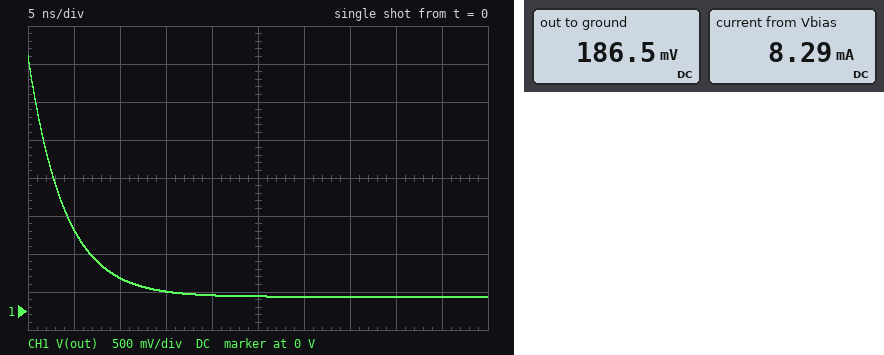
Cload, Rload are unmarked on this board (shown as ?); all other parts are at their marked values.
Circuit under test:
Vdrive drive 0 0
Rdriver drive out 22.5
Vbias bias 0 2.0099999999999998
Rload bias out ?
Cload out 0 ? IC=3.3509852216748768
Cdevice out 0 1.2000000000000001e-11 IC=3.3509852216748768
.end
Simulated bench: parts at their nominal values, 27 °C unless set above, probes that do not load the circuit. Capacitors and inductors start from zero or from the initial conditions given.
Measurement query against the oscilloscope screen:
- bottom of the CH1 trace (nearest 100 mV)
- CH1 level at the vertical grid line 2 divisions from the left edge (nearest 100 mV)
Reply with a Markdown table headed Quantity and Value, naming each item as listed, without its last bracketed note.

| Quantity | Value |
|---|---|
| bottom of the CH1 trace | 200 mV |
| CH1 level at the vertical grid line 2 divisions from the left edge | 400 mV |
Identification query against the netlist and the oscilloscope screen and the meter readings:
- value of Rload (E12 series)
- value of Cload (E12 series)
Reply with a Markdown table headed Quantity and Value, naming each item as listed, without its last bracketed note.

| Quantity | Value |
|---|---|
| value of Rload | 220 Ω |
| value of Cload | 180 pF |
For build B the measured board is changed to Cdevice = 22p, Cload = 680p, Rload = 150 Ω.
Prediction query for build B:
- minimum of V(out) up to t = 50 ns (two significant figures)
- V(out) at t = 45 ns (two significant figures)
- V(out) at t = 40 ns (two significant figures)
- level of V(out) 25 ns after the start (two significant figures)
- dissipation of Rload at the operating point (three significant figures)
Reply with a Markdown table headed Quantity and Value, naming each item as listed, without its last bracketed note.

| Quantity | Value |
|---|---|
| minimum of V(out) up to t = 50 ns | 340 mV |
| V(out) at t = 45 ns | 380 mV |
| V(out) at t = 40 ns | 430 mV |
| level of V(out) 25 ns after the start | 760 mV |
| dissipation of Rload at the operating point | 20.4 mW |
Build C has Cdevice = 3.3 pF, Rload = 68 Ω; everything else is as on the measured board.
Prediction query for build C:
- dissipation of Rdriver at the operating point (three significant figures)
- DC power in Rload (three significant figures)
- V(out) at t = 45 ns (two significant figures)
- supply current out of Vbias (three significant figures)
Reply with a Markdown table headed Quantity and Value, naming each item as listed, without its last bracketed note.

| Quantity | Value |
|---|---|
| dissipation of Rdriver at the operating point | 11.1 mW |
| DC power in Rload | 33.5 mW |
| V(out) at t = 45 ns | 500 mV |
| supply current out of Vbias | 22.2 mA |
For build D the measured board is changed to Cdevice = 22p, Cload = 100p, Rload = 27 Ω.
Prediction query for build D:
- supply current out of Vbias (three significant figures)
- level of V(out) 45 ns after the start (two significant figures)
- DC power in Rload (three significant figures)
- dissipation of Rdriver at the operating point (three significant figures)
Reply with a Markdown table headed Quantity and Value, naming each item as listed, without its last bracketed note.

| Quantity | Value |
|---|---|
| supply current out of Vbias | 40.6 mA |
| level of V(out) 45 ns after the start | 910 mV |
| DC power in Rload | 44.5 mW |
| dissipation of Rdriver at the operating point | 37.1 mW |
